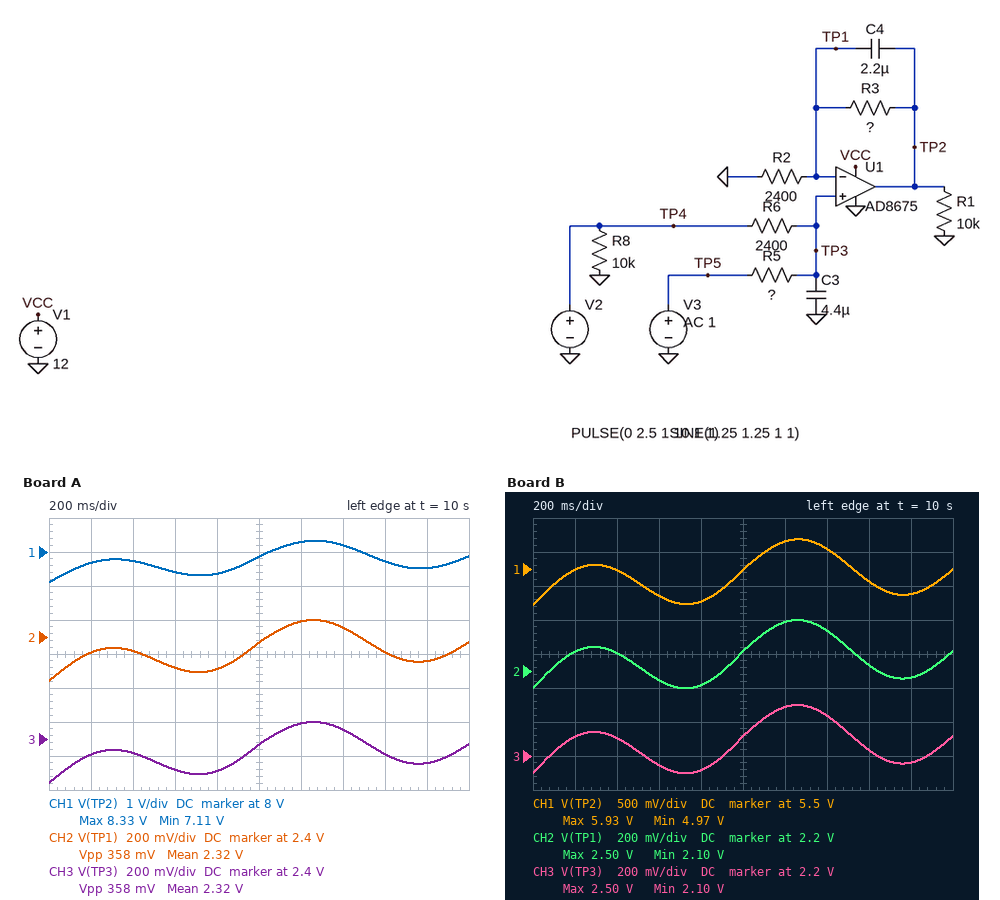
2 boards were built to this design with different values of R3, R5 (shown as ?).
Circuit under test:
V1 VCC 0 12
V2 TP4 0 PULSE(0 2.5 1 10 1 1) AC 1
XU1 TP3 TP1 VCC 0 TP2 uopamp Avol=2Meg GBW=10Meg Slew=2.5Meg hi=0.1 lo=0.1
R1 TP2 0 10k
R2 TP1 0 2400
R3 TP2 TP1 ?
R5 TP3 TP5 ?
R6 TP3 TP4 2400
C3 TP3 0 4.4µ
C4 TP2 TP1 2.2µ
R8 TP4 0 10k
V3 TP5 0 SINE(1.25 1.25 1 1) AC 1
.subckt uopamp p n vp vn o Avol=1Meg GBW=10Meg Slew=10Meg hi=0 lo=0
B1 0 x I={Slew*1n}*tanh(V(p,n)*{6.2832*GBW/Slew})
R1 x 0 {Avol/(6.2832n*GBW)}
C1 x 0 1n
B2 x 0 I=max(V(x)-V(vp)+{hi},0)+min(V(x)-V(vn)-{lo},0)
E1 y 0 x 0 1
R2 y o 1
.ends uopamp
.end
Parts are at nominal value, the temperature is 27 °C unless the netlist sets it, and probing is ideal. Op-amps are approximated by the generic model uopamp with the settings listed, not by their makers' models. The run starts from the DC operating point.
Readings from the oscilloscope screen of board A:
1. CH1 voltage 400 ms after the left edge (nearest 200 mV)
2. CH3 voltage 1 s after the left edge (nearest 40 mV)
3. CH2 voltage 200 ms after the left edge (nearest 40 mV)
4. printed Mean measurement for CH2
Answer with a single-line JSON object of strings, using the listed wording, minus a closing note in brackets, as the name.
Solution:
{"CH1 voltage 400 ms after the left edge": "7.8 V", "CH3 voltage 1 s after the left edge": "2.36 V", "CH2 voltage 200 ms after the left edge": "2.32 V", "printed Mean measurement for CH2": "2.32 V"}
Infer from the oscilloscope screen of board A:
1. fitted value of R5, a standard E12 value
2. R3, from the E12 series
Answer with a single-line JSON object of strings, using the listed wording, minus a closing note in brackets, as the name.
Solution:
{"fitted value of R5, a standard E12 value": "22 kΩ", "R3, from the E12 series": "5.6 kΩ"}
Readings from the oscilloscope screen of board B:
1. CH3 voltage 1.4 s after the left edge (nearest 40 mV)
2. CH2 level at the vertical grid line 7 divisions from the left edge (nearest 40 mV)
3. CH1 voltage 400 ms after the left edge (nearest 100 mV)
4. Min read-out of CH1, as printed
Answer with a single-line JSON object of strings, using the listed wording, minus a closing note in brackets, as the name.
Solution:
{"CH3 voltage 1.4 s after the left edge": "2.44 V", "CH2 level at the vertical grid line 7 divisions from the left edge": "2.44 V", "CH1 voltage 400 ms after the left edge": "5.5 V", "Min read-out of CH1, as printed": "4.97 V"}
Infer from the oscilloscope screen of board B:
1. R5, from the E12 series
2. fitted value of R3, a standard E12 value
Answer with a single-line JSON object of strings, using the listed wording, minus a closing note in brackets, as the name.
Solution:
{"R5, from the E12 series": "15 kΩ", "fitted value of R3, a standard E12 value": "3.3 kΩ"}
